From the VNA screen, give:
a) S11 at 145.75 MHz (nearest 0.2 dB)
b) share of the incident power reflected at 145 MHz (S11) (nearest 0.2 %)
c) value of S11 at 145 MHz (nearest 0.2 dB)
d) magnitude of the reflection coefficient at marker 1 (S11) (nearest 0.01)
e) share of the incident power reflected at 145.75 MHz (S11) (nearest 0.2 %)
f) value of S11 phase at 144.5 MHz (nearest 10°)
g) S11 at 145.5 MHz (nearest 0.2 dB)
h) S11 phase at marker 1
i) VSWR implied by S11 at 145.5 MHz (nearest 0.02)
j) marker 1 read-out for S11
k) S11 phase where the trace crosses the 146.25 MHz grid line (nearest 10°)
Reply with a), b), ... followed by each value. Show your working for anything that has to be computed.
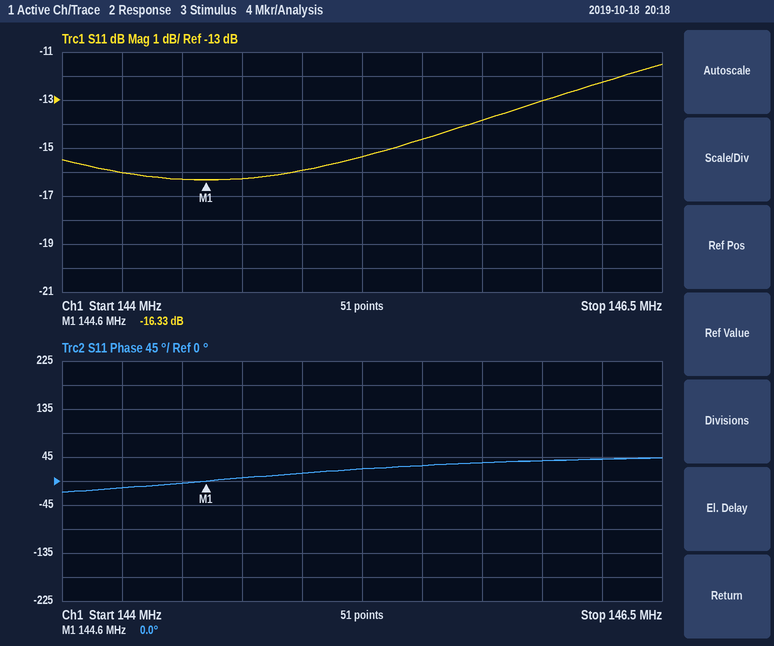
a) -13.8 dB
b) 10^(-16/10) ≈ 2.51 %, so 2.6 % to the nearest 0.2 %
c) -16.0 dB
d) 10^(-16.33/20) ≈ 0.15
e) 10^(-13.8/10) ≈ 4.2 %
f) 0°
g) -14.6 dB
h) 0.0°
i) |Γ| = 10^(-14.6/20) = 0.1862; VSWR = (1 + 0.1862)/(1 − 0.1862) ≈ 1.46
j) -16.33 dB
k) 40°
